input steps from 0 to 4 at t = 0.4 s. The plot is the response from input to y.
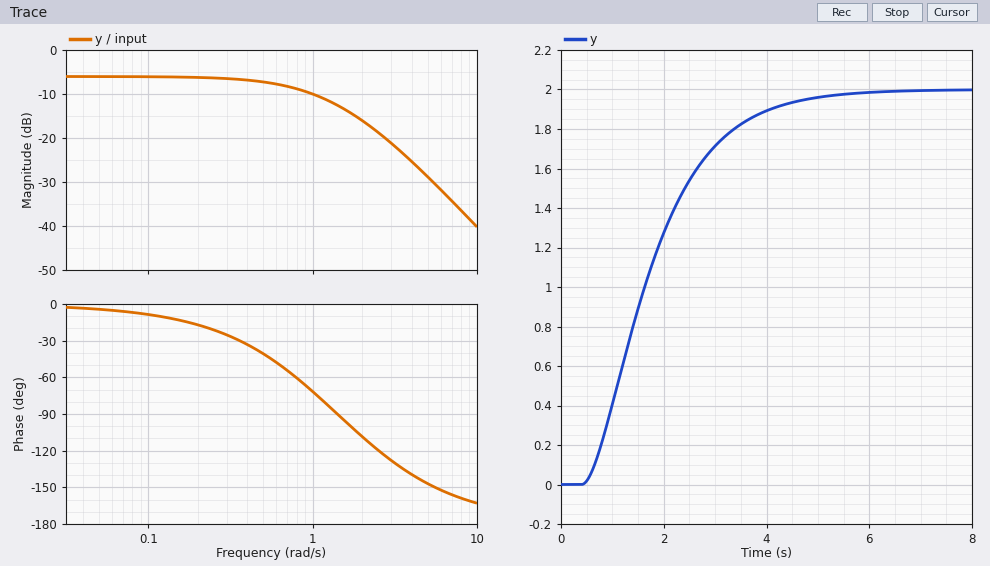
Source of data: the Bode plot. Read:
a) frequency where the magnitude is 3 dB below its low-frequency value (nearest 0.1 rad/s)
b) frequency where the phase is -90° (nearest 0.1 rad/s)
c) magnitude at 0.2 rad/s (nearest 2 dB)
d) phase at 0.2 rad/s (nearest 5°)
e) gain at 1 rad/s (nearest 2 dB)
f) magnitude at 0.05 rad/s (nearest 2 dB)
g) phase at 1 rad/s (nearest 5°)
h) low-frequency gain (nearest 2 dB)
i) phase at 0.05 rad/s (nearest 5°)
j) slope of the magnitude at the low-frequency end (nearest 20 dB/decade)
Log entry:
0.8 rad/s
1.4 rad/s
-6 dB
-15°
-10 dB
-6 dB
-70°
-6 dB
-5°
0 dB/decade
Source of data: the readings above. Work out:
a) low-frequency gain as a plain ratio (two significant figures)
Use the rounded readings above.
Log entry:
0.50
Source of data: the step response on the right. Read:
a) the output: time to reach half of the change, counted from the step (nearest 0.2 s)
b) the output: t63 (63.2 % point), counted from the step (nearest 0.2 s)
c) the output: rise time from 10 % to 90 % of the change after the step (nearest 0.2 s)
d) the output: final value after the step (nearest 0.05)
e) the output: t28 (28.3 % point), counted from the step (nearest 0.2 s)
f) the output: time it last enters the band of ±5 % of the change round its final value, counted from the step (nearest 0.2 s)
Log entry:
1.2 s
1.6 s
2.6 s
2.00
0.8 s
3.6 s
